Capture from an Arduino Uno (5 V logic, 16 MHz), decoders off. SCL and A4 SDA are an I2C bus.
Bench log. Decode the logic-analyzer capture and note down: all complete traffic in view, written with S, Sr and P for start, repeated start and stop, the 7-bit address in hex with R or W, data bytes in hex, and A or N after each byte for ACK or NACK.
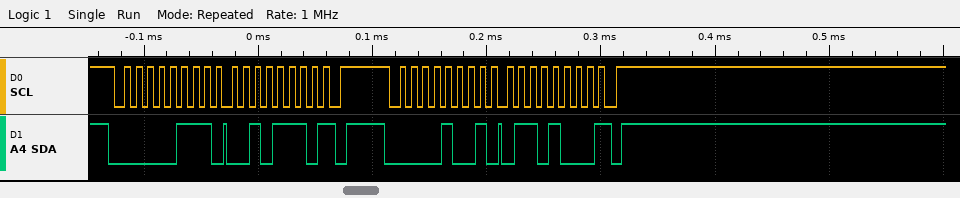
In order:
S 03R A 2E N P S 04R A 68 N P
